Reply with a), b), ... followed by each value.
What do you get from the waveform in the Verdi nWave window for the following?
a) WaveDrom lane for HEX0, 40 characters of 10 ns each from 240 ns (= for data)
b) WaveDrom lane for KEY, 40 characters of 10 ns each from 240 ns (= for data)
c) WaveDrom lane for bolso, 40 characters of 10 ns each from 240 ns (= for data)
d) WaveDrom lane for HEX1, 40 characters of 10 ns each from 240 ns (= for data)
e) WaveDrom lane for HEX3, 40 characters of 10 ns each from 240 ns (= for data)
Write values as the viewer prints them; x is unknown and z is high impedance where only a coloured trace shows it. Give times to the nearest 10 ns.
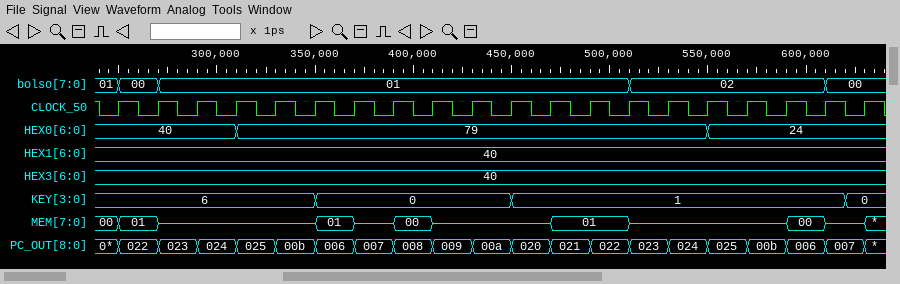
a) {name: 'HEX0', wave: '=......=.......................=........', data: '40 79 24'}
b) {name: 'KEY', wave: '=..........=.........=................=.', data: '6 0 1 0'}
c) {name: 'bolso', wave: '==.=.......................=.........=..', data: '01 00 01 02 00'}
d) {name: 'HEX1', wave: '=.......................................', data: '40'}
e) {name: 'HEX3', wave: '=.......................................', data: '40'}
